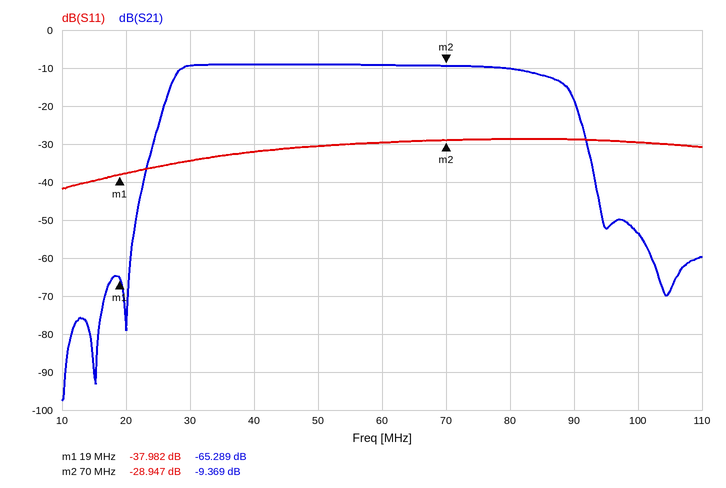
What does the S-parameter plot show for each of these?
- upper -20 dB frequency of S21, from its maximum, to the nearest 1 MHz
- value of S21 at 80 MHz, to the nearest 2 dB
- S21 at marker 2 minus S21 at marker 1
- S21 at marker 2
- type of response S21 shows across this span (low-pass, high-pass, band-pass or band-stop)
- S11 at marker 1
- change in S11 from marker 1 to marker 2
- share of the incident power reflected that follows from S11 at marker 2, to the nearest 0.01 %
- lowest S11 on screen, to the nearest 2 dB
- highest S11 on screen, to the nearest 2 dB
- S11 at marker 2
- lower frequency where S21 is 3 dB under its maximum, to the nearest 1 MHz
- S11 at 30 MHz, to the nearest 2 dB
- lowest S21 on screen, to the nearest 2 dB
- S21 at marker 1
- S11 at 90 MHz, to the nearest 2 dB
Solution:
92 MHz
-10 dB
55.920 dB
-9.369 dB
band-pass
-37.982 dB
9.035 dB
0.13 %
-42 dB
-28 dB
-28.947 dB
28 MHz
-34 dB
-98 dB
-65.289 dB
-28 dB
